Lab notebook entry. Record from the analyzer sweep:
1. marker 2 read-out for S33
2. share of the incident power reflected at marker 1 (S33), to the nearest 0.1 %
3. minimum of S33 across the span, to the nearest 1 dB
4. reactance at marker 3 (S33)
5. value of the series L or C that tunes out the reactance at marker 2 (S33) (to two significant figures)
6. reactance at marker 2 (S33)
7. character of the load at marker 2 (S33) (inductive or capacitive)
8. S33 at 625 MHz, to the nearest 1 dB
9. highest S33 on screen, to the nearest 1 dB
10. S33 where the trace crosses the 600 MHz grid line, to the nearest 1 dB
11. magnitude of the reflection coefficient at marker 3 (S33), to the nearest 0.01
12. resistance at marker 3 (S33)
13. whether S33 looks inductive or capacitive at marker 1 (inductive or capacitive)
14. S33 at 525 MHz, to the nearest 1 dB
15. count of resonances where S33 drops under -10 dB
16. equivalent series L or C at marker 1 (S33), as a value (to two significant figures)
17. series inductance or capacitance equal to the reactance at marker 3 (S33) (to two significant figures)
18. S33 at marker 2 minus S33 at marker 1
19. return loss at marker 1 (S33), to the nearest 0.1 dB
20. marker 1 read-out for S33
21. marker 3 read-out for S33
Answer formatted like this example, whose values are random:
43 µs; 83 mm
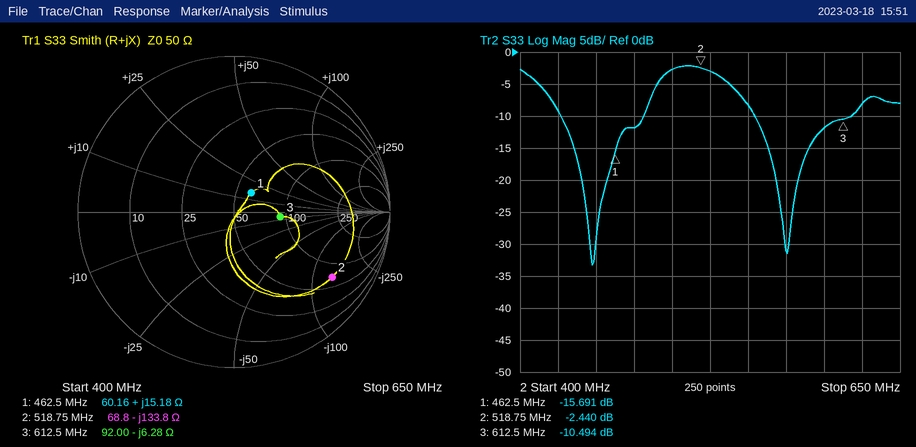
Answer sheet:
-2.440 dB; 2.7 %; -33 dB; -6.28 Ω; 41 nH; -133.8 Ω; capacitive; -8 dB; -2 dB; -12 dB; 0.30; 92.00 Ω; inductive; -3 dB; 2; 5.2 nH; 41 pF; 13.251 dB; 15.7 dB; -15.691 dB; -10.494 dB
